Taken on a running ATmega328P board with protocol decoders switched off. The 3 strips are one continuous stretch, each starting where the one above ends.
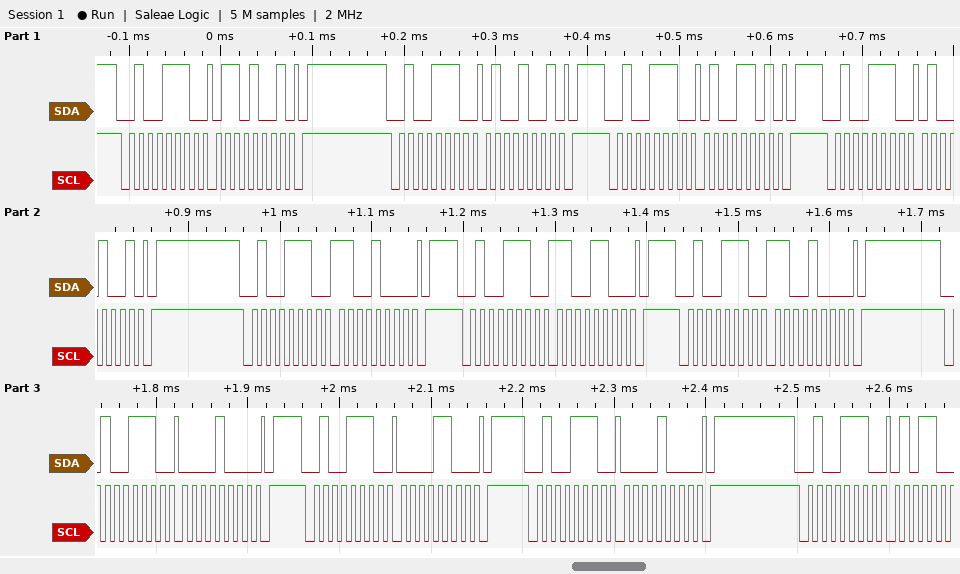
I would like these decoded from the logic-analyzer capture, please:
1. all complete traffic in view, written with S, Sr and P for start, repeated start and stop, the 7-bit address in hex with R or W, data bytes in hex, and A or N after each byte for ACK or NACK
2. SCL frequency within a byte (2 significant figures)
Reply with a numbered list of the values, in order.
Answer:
1. S 27W A 69 A P S 27W A 49 A P S 27W A 4D A P S 27W A 49 A P S 27W A C8 A P S 27W A CC A P S 27W A C8 A P S 27W A 08 A P S 27W A 0C A P S 27W A 08 A P S 27W A
2. 100 kHz
